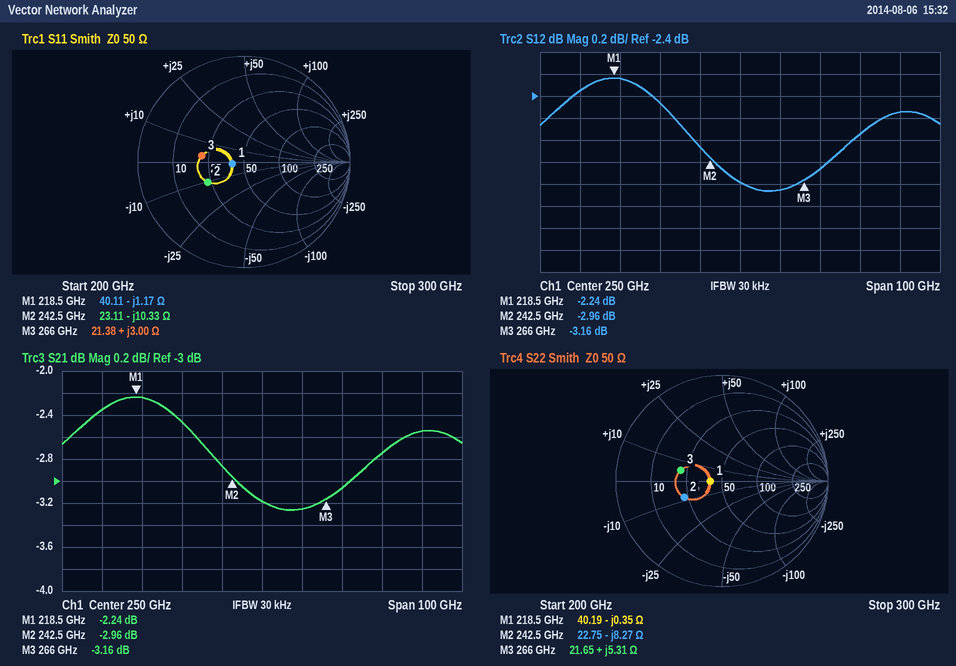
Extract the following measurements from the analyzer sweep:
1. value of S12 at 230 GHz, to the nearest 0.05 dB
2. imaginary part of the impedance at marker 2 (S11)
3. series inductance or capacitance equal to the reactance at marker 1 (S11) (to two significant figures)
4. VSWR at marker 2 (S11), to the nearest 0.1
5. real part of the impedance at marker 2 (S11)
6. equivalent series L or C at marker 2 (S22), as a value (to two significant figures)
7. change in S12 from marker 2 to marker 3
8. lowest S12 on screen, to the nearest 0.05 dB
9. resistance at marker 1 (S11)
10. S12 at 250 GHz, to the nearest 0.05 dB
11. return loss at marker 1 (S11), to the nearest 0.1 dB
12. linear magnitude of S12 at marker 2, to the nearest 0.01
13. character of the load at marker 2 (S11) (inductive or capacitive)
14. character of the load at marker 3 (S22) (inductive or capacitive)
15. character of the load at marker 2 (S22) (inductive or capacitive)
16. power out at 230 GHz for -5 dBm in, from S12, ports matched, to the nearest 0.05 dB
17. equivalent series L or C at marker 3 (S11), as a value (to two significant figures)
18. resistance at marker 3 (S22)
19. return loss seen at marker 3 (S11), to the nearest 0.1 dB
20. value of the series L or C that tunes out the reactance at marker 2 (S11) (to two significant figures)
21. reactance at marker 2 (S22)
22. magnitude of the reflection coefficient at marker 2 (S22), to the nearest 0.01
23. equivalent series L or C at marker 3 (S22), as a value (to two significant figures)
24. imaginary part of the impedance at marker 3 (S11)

-2.45 dB
-10.33 Ω
620 fF
2.3
23.11 Ω
79 fF
-0.20 dB
-3.25 dB
40.11 Ω
-3.20 dB
19.1 dB
0.71
capacitive
inductive
capacitive
-7.45 dBm
1.8 pH
21.65 Ω
7.9 dB
6.8 pH
-8.27 Ω
0.39
3.2 pH
+3.00 Ω
